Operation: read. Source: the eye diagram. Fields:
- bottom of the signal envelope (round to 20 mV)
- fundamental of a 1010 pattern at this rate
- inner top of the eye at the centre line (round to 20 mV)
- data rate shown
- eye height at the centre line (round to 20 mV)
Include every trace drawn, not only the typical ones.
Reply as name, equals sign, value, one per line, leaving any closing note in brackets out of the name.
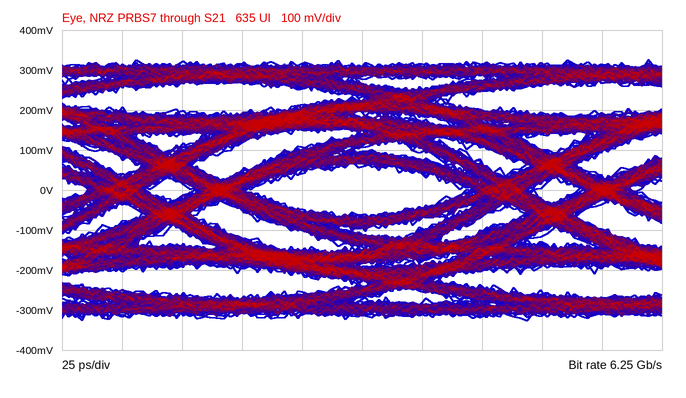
bottom of the signal envelope = -320 mV
fundamental of a 1010 pattern at this rate = 3.125 GHz
inner top of the eye at the centre line = 60 mV
data rate shown = 6.25 Gb/s
eye height at the centre line = 120 mV
